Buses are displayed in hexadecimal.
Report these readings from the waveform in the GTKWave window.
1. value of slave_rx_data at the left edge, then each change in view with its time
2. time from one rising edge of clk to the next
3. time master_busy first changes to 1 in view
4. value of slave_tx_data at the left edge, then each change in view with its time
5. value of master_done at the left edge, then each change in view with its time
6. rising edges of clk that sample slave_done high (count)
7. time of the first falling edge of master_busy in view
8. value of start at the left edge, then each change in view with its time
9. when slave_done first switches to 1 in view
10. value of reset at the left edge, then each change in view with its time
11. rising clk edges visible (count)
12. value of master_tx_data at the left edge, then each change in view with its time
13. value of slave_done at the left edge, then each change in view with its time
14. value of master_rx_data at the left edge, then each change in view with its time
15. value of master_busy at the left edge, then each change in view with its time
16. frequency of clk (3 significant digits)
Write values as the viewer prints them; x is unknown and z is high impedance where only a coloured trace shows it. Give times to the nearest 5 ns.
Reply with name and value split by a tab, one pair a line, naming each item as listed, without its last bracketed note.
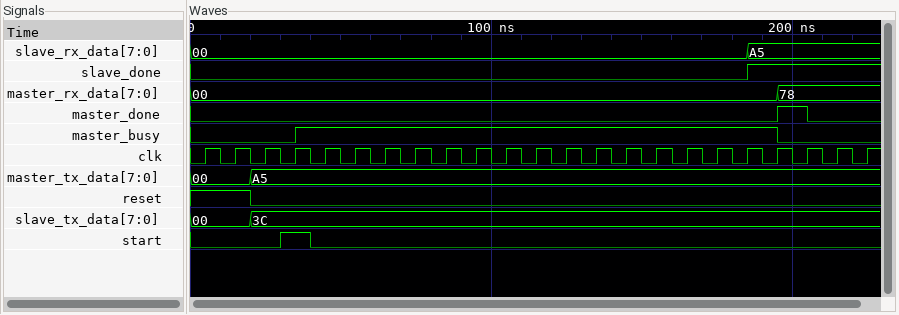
value of slave_rx_data at the left edge, then each change in view with its time	00, A5 at 185 ns
time from one rising edge of clk to the next	10 ns
time master_busy first changes to 1 in view	35 ns
value of slave_tx_data at the left edge, then each change in view with its time	00, 3C at 20 ns
value of master_done at the left edge, then each change in view with its time	0, 1 at 195 ns, 0 at 205 ns
rising edges of clk that sample slave_done high	4
time of the first falling edge of master_busy in view	195 ns
value of start at the left edge, then each change in view with its time	0, 1 at 30 ns, 0 at 40 ns
when slave_done first switches to 1 in view	185 ns
value of reset at the left edge, then each change in view with its time	1, 0 at 20 ns
rising clk edges visible	23
value of master_tx_data at the left edge, then each change in view with its time	00, A5 at 20 ns
value of slave_done at the left edge, then each change in view with its time	0, 1 at 185 ns
value of master_rx_data at the left edge, then each change in view with its time	00, 78 at 195 ns
value of master_busy at the left edge, then each change in view with its time	0, 1 at 35 ns, 0 at 195 ns
frequency of clk	100 MHz
